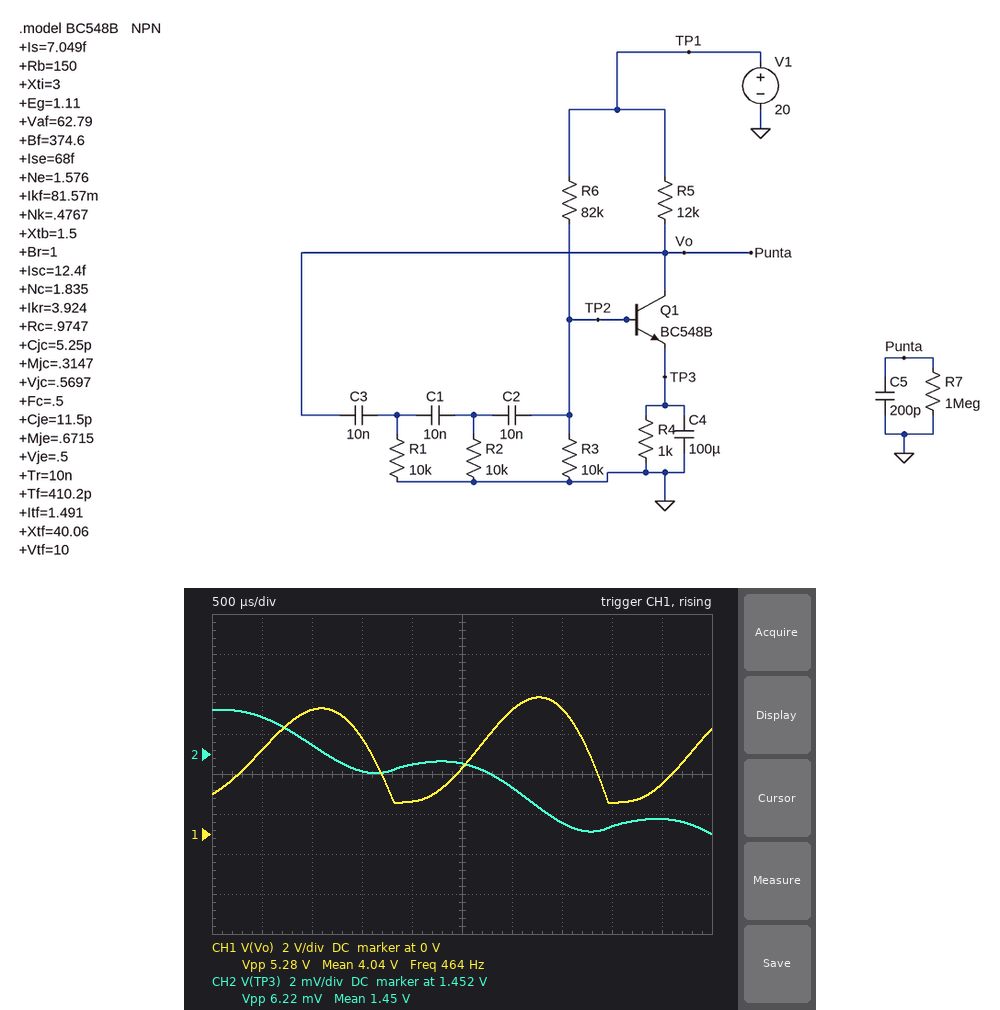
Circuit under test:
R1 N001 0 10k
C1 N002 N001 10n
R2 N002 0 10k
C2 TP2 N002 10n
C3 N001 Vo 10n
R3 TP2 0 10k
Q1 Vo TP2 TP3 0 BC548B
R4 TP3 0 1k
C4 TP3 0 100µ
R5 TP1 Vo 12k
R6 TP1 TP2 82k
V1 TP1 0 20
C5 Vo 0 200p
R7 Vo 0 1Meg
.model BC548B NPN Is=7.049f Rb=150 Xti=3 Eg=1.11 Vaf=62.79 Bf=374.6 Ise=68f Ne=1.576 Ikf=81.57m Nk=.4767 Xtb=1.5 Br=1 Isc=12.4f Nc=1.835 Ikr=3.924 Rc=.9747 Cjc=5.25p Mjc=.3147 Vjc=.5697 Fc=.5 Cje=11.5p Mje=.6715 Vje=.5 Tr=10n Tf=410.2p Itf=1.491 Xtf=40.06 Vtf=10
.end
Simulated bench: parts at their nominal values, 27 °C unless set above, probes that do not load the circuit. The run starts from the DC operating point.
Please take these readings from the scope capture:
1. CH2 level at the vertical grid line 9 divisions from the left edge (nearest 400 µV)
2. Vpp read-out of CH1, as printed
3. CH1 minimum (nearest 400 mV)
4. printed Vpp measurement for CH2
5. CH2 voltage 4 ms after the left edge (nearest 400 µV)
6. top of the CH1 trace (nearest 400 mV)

1.4488 V
5.28 V
1.6 V
6.22 mV
1.4484 V
6.8 V
